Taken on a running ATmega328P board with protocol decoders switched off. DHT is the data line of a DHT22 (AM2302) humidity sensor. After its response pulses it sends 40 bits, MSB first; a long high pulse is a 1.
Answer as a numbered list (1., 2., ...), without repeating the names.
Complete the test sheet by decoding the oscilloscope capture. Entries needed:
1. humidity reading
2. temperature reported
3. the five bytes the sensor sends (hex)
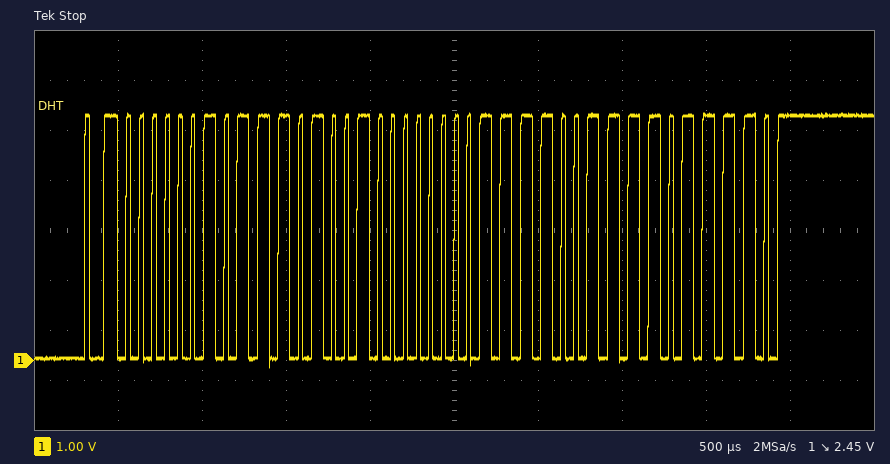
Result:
1. 74.5 %
2. 24.3 °C
3. 02 E9 00 F3 DE
